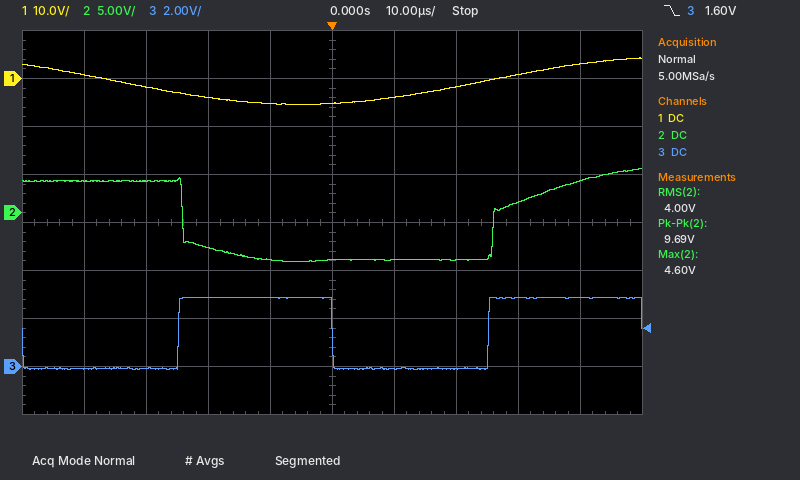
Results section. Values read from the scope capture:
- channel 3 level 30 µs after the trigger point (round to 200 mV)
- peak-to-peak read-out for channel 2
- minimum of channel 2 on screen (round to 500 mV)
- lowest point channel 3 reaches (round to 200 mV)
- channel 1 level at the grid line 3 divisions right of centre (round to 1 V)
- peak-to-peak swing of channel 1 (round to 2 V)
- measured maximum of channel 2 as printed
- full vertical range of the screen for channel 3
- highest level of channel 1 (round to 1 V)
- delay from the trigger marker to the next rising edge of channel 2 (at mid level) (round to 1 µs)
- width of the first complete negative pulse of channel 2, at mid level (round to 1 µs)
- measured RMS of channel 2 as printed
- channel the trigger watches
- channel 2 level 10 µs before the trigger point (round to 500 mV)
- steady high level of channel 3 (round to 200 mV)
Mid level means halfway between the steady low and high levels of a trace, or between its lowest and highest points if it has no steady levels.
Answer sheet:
2.8 V
9.69 V
-5.0 V
-200 mV
1 V
10 V
4.60 V
16 V
4 V
26 µs
50 µs
4.00 V
channel 3
-5.0 V
2.8 V
